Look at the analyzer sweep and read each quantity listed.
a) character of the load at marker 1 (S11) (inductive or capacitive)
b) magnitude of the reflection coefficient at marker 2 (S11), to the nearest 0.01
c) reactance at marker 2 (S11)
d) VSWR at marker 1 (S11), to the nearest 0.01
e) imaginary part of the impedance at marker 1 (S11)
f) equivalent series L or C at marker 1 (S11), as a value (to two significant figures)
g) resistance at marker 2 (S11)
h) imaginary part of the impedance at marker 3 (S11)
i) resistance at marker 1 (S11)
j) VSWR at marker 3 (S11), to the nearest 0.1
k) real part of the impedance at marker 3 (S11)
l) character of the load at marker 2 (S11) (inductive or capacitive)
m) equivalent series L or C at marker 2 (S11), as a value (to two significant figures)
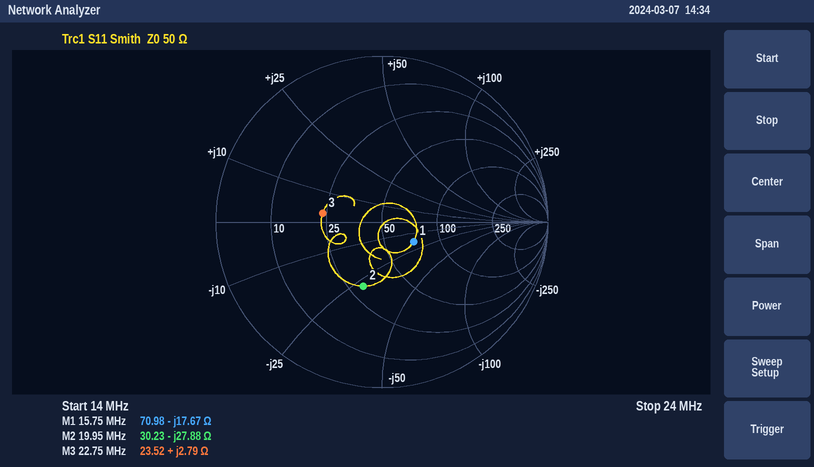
capacitive
0.40
-27.88 Ω
1.58
-17.67 Ω
570 pF
30.23 Ω
+2.79 Ω
70.98 Ω
2.1
23.52 Ω
capacitive
290 pF
